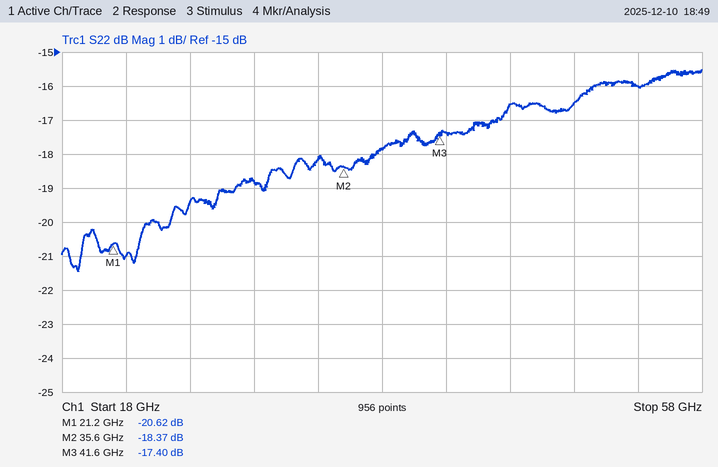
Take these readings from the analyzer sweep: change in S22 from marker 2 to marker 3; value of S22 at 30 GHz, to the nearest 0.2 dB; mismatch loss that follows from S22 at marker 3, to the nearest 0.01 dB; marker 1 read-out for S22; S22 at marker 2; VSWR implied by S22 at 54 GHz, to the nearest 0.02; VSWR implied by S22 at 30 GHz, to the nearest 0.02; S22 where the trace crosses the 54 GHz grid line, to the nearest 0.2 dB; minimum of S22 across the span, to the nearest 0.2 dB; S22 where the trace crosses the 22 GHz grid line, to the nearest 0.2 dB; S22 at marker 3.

0.97 dB
-18.8 dB
0.08 dB
-20.62 dB
-18.37 dB
1.38
1.26
-16.0 dB
-21.4 dB
-21.0 dB
-17.40 dB
